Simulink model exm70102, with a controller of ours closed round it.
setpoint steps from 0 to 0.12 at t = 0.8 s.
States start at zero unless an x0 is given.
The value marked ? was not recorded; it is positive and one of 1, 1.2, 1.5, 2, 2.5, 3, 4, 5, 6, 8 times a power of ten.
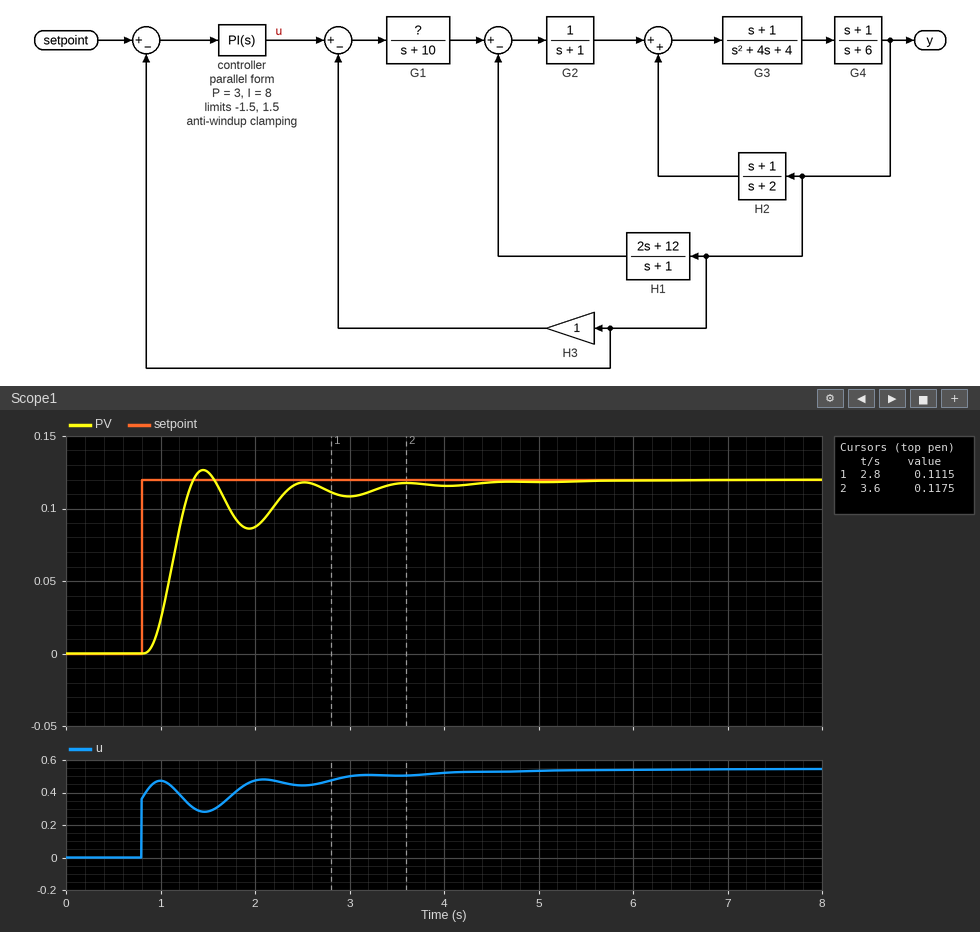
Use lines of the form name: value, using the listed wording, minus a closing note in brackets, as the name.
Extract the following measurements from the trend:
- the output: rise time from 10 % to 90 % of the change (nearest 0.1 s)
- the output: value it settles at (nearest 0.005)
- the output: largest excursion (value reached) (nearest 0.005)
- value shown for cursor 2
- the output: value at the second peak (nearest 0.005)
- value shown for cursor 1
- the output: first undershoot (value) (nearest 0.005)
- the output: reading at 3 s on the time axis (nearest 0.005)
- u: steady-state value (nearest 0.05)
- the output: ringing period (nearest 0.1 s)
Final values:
the output: rise time from 10 % to 90 % of the change: 0.3 s
the output: value it settles at: 0.120
the output: largest excursion (value reached): 0.125
value shown for cursor 2: 0.1175
the output: value at the second peak: 0.120
value shown for cursor 1: 0.1115
the output: first undershoot (value): 0.085
the output: reading at 3 s on the time axis: 0.110
u: steady-state value: 0.55
the output: ringing period: 1.1 s
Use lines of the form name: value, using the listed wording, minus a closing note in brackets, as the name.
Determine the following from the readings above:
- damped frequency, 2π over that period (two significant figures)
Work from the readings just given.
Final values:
damped frequency, 2π over that period: 5.7 rad/s
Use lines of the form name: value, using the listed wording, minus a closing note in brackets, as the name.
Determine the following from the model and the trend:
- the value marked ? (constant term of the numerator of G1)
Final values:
the value marked ?: 100
